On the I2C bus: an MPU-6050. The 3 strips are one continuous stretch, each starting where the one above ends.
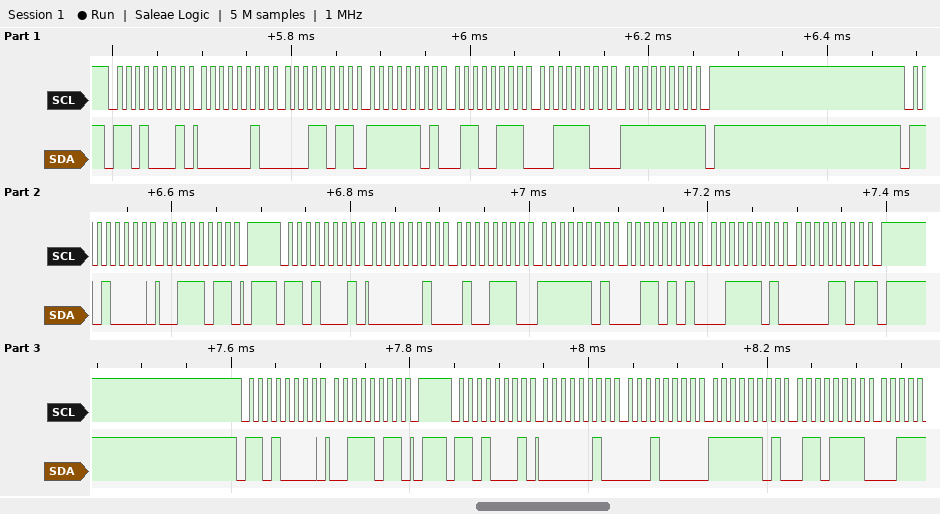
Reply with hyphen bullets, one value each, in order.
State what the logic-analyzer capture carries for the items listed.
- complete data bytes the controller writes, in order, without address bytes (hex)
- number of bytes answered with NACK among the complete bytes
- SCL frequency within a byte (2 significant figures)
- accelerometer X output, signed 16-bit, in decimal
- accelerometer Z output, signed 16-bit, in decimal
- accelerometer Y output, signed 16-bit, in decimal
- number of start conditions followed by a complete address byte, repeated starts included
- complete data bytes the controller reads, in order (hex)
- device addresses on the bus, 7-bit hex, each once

- 3B 3B
- 2
- 100 kHz
- 590
- 15629
- -715
- 5
- 02 1B FD 67 3C FF 02 4E FD 35 3D 0D 02 10 FD 6F
- 0x68
